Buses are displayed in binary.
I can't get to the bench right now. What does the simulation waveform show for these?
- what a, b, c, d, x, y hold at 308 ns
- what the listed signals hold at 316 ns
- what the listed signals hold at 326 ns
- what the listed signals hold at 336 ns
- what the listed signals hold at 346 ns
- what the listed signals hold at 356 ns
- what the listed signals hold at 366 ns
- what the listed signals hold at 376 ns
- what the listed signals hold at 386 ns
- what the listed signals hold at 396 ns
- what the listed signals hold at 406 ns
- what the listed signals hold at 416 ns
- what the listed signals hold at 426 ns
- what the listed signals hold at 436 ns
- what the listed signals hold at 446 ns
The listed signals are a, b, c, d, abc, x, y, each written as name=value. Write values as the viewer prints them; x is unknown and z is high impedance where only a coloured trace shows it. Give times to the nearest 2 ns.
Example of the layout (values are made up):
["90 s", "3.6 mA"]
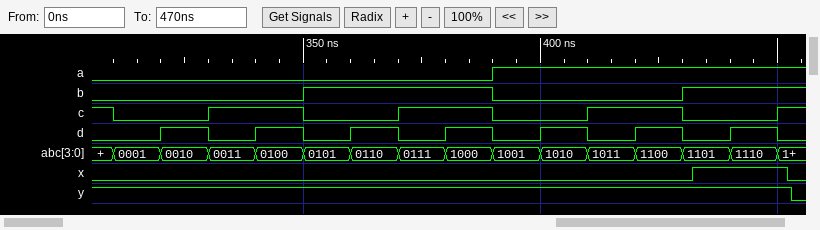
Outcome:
["a=0, b=0, c=1, d=0, x=0, y=1", "a=0, b=0, c=0, d=0, abc=0001, x=0, y=1", "a=0, b=0, c=0, d=1, abc=0010, x=0, y=1", "a=0, b=0, c=1, d=0, abc=0011, x=0, y=1", "a=0, b=0, c=1, d=1, abc=0100, x=0, y=1", "a=0, b=1, c=0, d=0, abc=0101, x=0, y=1", "a=0, b=1, c=0, d=1, abc=0110, x=0, y=1", "a=0, b=1, c=1, d=0, abc=0111, x=0, y=1", "a=0, b=1, c=1, d=1, abc=1000, x=0, y=1", "a=1, b=0, c=0, d=0, abc=1001, x=0, y=1", "a=1, b=0, c=0, d=1, abc=1010, x=0, y=1", "a=1, b=0, c=1, d=0, abc=1011, x=0, y=1", "a=1, b=0, c=1, d=1, abc=1100, x=0, y=1", "a=1, b=1, c=0, d=0, abc=1101, x=1, y=1", "a=1, b=1, c=0, d=1, abc=1110, x=1, y=1"]
